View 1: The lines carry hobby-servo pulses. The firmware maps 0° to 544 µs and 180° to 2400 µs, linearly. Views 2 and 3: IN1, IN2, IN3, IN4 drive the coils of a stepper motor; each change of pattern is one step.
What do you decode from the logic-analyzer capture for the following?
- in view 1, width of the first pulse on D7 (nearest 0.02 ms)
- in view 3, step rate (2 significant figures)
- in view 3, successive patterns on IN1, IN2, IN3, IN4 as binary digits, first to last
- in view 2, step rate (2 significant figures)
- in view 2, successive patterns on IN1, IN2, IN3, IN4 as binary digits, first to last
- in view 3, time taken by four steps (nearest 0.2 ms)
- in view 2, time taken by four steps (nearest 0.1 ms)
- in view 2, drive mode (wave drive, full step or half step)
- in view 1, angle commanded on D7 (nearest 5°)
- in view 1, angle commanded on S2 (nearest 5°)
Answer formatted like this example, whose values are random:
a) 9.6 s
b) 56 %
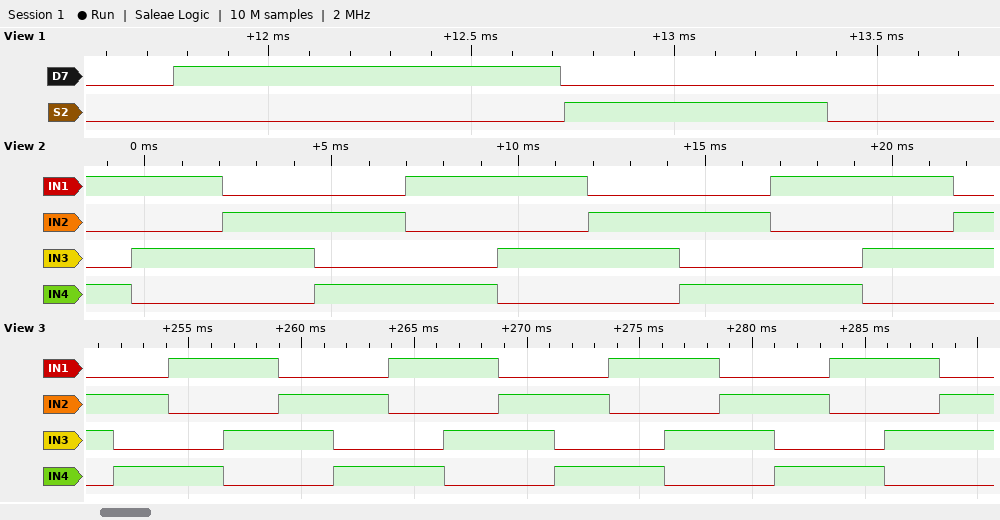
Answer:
a) 0.96 ms
b) 410 steps/s
c) 0110 0101 1001 1010 0110 0101 1001 1010 0110 0101 1001 1010 0110 0101 1001 1010 0110
d) 410 steps/s
e) 1001 1010 0110 0101 1001 1010 0110 0101 1001 1010 0110
f) 9.8 ms
g) 9.8 ms
h) full step
i) 40°
j) 10°
